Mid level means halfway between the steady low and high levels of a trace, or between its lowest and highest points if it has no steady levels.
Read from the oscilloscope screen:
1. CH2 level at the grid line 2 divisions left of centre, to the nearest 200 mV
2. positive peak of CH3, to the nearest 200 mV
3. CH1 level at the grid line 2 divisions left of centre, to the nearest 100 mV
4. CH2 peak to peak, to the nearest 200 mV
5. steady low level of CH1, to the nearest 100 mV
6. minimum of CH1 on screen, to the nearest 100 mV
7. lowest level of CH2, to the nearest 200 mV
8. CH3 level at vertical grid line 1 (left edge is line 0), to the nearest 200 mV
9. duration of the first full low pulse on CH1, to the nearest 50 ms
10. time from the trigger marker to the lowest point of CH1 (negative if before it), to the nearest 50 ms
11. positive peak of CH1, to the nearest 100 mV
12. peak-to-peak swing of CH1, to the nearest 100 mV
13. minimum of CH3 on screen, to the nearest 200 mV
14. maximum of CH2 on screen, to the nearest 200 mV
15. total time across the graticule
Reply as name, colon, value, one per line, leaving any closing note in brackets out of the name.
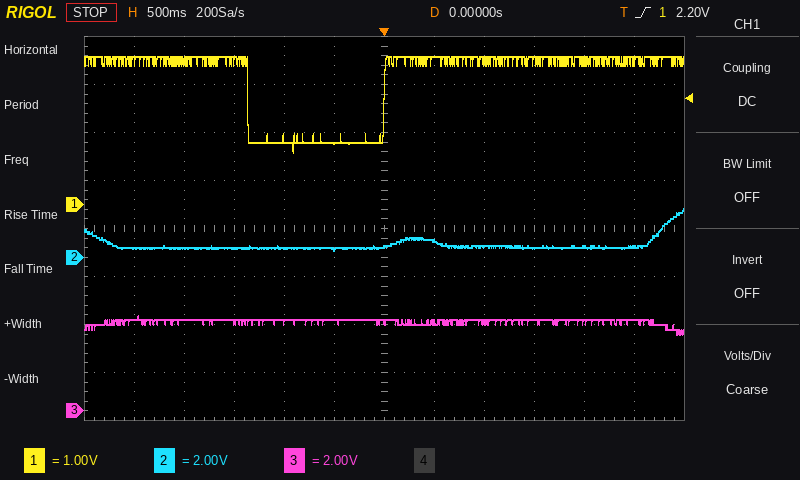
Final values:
CH2 level at the grid line 2 divisions left of centre, to the nearest 200 mV: 400 mV
positive peak of CH3, to the nearest 200 mV: 4.0 V
CH1 level at the grid line 2 divisions left of centre, to the nearest 100 mV: 1.4 V
CH2 peak to peak, to the nearest 200 mV: 1.8 V
steady low level of CH1, to the nearest 100 mV: 1.3 V
minimum of CH1 on screen, to the nearest 100 mV: 1.1 V
lowest level of CH2, to the nearest 200 mV: 200 mV
CH3 level at vertical grid line 1 (left edge is line 0), to the nearest 200 mV: 3.8 V
duration of the first full low pulse on CH1, to the nearest 50 ms: 1.35 s
time from the trigger marker to the lowest point of CH1 (negative if before it), to the nearest 50 ms: -900 ms
positive peak of CH1, to the nearest 100 mV: 3.1 V
peak-to-peak swing of CH1, to the nearest 100 mV: 2.0 V
minimum of CH3 on screen, to the nearest 200 mV: 3.2 V
maximum of CH2 on screen, to the nearest 200 mV: 2.0 V
total time across the graticule: 6 s
